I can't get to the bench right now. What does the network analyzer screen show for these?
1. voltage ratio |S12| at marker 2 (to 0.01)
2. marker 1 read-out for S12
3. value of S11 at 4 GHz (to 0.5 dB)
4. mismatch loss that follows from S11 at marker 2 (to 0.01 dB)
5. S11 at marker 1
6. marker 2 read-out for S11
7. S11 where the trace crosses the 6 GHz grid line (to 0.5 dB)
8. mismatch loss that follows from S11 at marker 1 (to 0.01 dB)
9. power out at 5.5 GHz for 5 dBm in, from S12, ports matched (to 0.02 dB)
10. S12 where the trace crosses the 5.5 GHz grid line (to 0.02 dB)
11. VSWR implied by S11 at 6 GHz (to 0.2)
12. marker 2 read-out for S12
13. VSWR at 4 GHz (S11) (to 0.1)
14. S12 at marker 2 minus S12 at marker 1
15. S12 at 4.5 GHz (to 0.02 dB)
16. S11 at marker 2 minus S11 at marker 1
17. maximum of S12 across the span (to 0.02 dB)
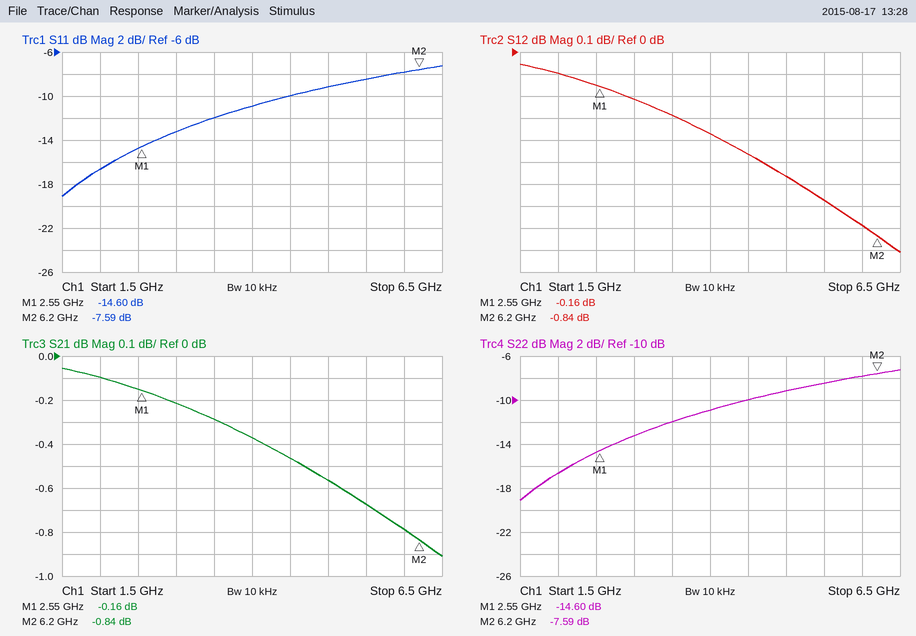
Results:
0.91
-0.16 dB
-11.0 dB
0.83 dB
-14.60 dB
-7.59 dB
-8.0 dB
0.15 dB
4.32 dBm
-0.68 dB
2.4
-0.84 dB
1.8
-0.68 dB
-0.46 dB
7.01 dB
-0.06 dB
